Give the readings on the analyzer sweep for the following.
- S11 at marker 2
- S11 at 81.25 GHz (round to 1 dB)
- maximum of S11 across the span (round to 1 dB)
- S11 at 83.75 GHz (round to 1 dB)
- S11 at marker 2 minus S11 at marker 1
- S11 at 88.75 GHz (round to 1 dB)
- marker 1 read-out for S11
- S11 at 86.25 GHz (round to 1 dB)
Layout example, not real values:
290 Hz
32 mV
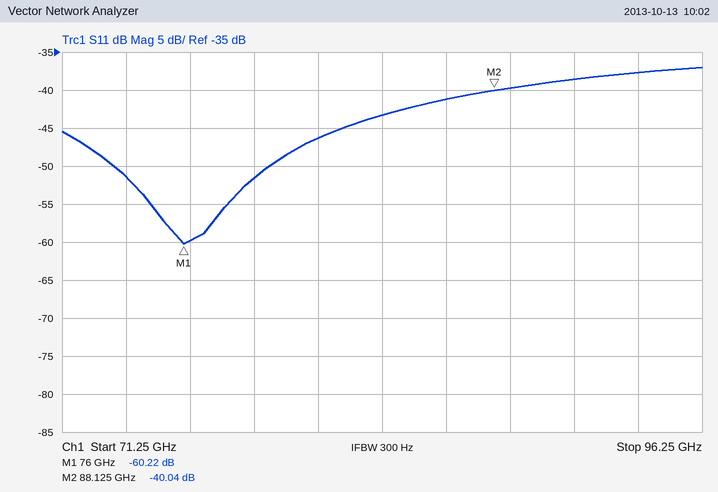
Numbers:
-40.04 dB
-46 dB
-37 dB
-43 dB
20.18 dB
-40 dB
-60.22 dB
-41 dB
